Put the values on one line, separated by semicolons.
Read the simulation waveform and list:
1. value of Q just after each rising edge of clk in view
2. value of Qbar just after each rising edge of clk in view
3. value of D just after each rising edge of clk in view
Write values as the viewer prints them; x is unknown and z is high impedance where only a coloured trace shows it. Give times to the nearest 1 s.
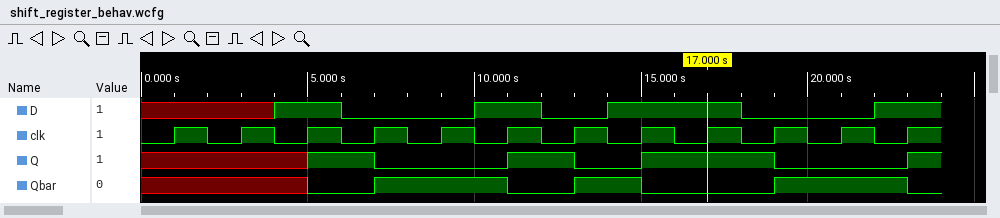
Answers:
x x 1 0 0 1 0 1 1 0 0 1; x x 0 1 1 0 1 0 0 1 1 0; x x 1 0 0 1 0 1 1 0 0 1
